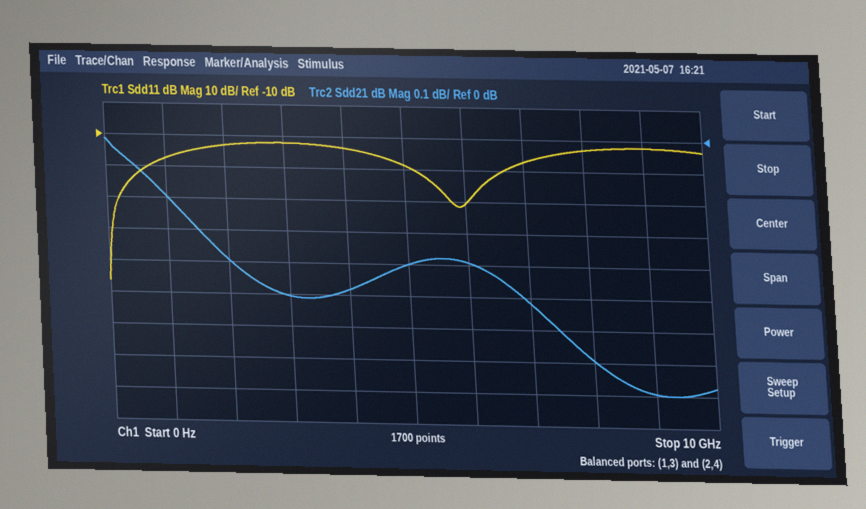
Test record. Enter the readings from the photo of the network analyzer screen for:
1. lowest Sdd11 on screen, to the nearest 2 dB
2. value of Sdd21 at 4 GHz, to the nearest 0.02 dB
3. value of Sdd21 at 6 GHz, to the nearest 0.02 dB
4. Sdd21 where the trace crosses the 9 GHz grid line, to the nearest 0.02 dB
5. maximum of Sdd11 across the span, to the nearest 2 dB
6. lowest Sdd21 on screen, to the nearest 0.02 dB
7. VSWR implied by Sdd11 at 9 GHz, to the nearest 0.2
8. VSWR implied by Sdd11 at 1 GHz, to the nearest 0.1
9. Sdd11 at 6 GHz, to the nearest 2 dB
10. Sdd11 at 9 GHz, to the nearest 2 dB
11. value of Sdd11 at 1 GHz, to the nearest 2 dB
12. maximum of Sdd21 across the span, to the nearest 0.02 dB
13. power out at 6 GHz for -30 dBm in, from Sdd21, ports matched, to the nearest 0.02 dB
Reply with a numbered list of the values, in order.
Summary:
1. -56 dB
2. -0.48 dB
3. -0.40 dB
4. -0.80 dB
5. -12 dB
6. -0.80 dB
7. 1.6
8. 1.3
9. -30 dB
10. -12 dB
11. -18 dB
12. -0.02 dB
13. -30.40 dBm
